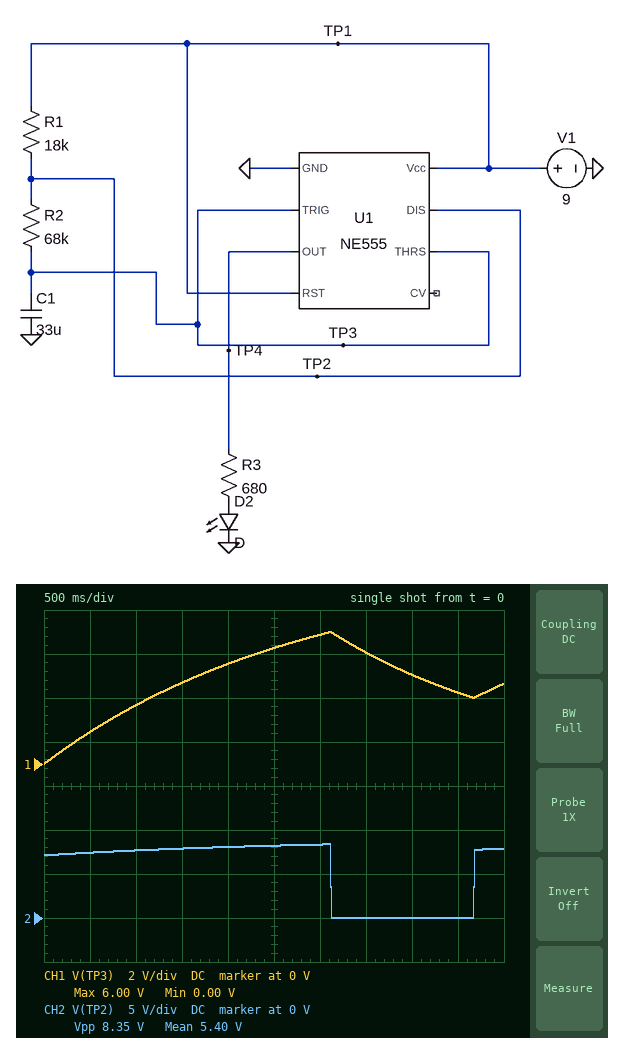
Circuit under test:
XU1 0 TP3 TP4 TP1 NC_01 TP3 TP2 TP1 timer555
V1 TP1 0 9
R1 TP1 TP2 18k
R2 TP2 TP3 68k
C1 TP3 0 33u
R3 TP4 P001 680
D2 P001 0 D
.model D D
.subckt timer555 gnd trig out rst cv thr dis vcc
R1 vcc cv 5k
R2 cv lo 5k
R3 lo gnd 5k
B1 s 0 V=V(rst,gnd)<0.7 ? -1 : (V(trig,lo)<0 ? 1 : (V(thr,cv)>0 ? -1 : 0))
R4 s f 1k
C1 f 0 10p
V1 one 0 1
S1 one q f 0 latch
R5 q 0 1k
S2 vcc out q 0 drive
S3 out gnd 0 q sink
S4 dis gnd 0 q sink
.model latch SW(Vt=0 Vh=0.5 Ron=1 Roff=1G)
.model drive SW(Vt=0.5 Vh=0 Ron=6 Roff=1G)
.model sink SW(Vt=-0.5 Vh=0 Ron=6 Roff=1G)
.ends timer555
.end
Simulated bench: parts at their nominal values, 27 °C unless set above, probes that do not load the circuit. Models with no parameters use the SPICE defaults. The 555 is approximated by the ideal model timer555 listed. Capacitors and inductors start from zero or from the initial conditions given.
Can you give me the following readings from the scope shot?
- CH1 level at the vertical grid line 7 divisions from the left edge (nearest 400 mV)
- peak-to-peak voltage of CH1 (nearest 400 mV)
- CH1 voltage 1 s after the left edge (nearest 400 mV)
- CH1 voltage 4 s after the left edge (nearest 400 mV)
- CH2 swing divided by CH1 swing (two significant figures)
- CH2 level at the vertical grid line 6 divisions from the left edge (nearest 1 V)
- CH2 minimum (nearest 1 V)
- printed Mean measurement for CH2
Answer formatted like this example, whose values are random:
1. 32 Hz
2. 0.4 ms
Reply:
1. 5.2 V
2. 6.0 V
3. 2.8 V
4. 4.0 V
5. 1.4
6. 8 V
7. 0 V
8. 5.40 V
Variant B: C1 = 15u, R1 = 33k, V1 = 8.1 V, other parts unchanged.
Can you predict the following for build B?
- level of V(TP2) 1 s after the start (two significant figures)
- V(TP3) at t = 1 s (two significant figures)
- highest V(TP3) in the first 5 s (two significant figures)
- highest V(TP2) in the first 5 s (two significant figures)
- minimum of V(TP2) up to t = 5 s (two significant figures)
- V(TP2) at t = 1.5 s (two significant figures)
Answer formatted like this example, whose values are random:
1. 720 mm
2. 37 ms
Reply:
1. 6.7 V
2. 3.9 V
3. 5.4 V
4. 7.2 V
5. 1.7 mV
6. 7.1 V
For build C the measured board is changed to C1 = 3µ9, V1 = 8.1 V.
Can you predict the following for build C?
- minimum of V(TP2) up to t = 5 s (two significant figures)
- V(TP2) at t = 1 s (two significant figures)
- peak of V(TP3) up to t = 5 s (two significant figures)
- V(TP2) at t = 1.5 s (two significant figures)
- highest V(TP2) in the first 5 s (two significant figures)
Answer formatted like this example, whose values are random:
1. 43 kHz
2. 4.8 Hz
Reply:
1. 2.9 mV
2. 7.1 V
3. 5.4 V
4. 7.3 V
5. 7.5 V
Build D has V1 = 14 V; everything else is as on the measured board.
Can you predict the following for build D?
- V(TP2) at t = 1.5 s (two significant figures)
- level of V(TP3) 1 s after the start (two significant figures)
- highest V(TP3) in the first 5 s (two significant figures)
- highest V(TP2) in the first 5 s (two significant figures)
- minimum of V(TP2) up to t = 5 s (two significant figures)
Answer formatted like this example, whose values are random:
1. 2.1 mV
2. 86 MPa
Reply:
1. 12 V
2. 4.2 V
3. 9.3 V
4. 13 V
5. 5.1 mV
